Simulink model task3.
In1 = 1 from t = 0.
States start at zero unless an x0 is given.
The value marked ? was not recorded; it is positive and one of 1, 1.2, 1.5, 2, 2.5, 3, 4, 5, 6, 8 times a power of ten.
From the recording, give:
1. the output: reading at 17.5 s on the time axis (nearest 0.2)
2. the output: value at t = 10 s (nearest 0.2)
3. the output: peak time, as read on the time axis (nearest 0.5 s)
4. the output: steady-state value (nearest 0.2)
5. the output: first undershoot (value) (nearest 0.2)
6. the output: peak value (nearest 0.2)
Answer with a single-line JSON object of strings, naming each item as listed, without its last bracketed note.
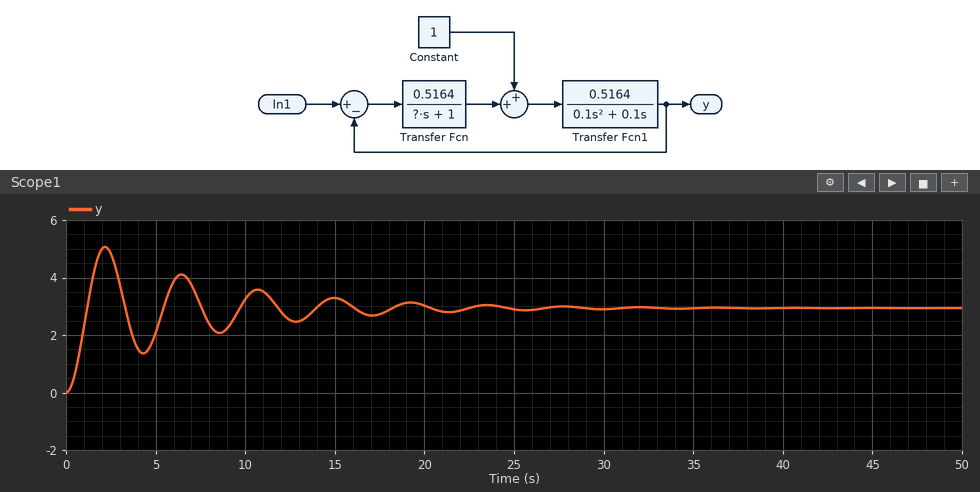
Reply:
{"the output: reading at 17.5 s on the time axis": "2.8", "the output: value at t = 10 s": "3.2", "the output: peak time, as read on the time axis": "2.0 s", "the output: steady-state value": "3.0", "the output: first undershoot (value)": "1.4", "the output: peak value": "5.0"}
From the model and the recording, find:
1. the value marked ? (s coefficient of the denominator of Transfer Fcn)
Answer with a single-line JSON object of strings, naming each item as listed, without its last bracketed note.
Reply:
{"the value marked ?": "0.3"}
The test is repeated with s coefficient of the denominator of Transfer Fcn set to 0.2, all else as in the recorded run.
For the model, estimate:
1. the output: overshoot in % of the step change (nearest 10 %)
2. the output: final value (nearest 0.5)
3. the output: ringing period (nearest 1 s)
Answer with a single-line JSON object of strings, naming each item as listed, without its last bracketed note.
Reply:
{"the output: overshoot in % of the step change": "60 %", "the output: final value": "3.0", "the output: ringing period": "4 s"}
